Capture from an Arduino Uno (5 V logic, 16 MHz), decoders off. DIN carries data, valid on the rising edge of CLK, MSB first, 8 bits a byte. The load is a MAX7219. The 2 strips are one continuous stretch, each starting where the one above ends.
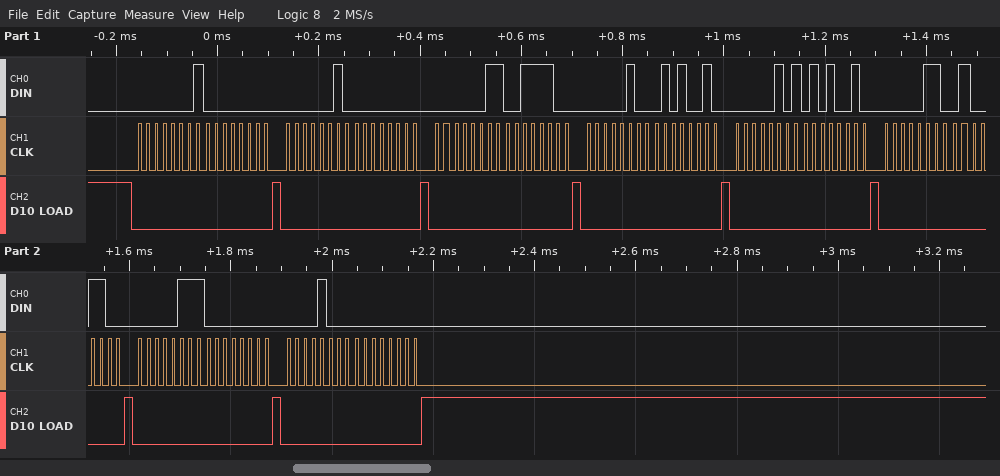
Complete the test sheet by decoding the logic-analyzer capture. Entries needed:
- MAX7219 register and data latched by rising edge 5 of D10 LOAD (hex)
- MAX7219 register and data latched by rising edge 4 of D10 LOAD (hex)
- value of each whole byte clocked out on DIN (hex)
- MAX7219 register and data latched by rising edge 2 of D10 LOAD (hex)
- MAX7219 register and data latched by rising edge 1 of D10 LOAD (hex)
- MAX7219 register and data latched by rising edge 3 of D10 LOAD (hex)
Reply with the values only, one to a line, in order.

register 0x5, data 0x52
register 0x4, data 0x52
01 00 02 00 03 3C 04 52 05 52 06 4C 07 00 08 00
register 0x2, data 0x00
register 0x1, data 0x00
register 0x3, data 0x3C
